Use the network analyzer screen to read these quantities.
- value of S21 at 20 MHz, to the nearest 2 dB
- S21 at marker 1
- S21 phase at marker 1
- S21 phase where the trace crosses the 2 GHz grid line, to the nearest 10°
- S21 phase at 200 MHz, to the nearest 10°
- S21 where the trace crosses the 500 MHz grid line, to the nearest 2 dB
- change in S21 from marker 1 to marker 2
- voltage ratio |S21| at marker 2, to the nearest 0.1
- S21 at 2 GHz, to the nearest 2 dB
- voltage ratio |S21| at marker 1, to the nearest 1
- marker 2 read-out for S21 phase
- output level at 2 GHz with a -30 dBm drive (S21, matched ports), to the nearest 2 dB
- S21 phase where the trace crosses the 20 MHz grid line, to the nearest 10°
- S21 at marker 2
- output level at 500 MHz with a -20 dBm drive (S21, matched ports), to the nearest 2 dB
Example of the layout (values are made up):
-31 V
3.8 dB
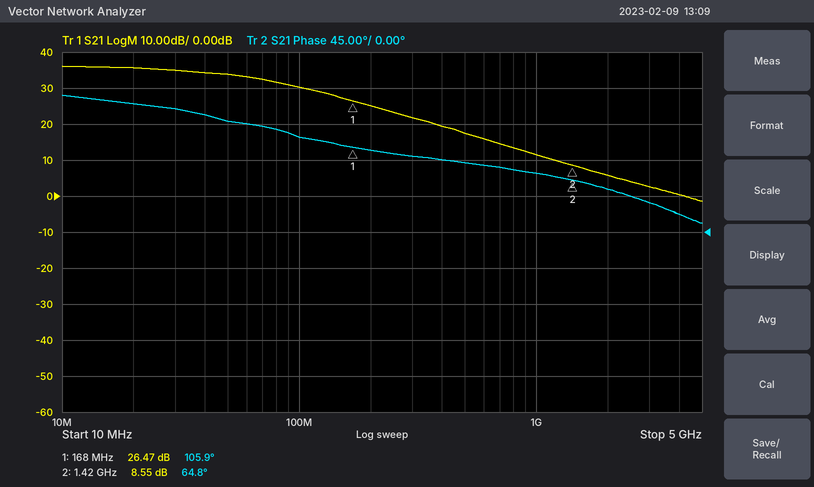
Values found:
36 dB
26.47 dB
105.9°
50°
100°
18 dB
-17.92 dB
2.7
6 dB
21
64.8°
-24 dBm
160°
8.55 dB
-2 dBm
